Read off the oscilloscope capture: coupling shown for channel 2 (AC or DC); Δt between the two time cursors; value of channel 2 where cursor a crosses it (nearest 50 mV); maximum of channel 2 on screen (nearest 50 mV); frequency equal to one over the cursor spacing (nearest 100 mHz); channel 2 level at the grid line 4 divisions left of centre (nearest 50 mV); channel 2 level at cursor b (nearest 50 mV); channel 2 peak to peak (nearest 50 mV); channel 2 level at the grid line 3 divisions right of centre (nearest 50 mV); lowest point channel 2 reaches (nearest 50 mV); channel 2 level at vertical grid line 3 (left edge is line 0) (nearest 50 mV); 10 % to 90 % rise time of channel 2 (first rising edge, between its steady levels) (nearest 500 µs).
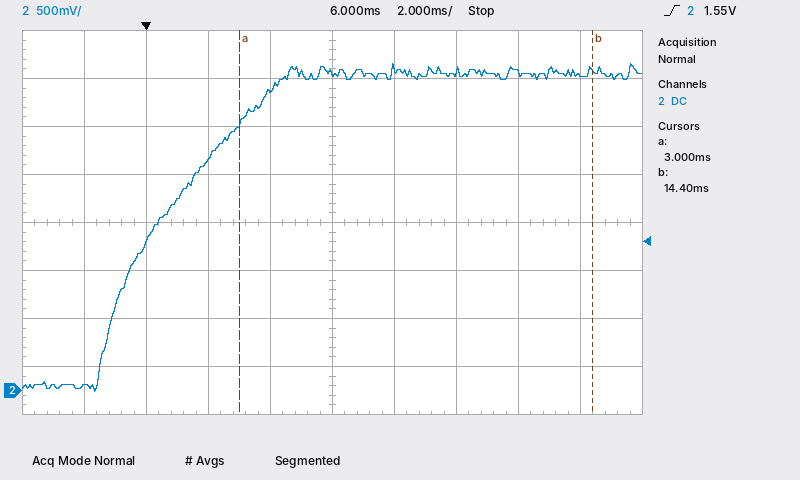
DC
11.4 ms
2.80 V
3.40 V
87.7 Hz
50 mV
3.35 V
3.40 V
3.30 V
0 mV
2.40 V
5.0 ms
